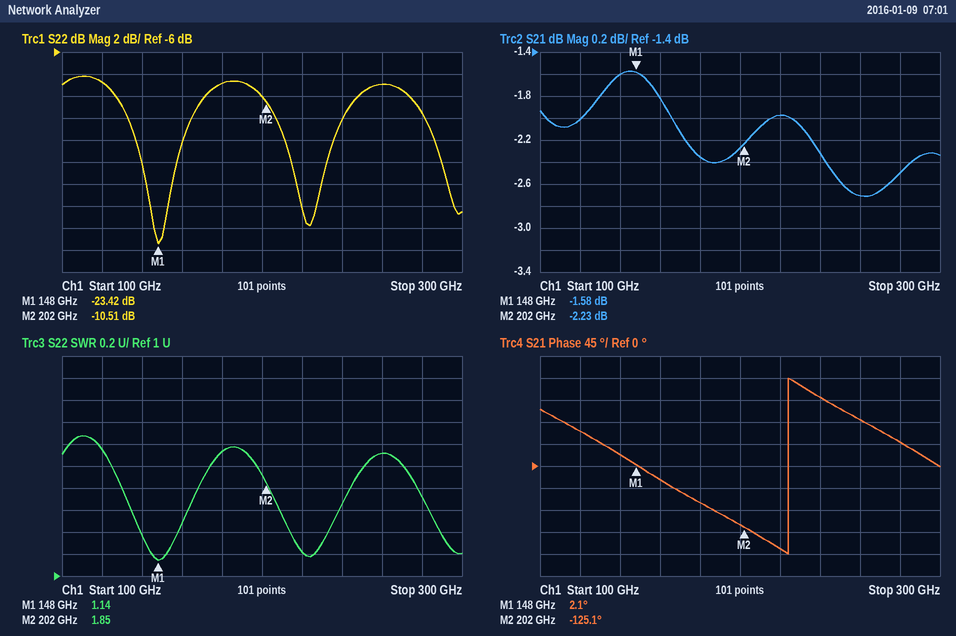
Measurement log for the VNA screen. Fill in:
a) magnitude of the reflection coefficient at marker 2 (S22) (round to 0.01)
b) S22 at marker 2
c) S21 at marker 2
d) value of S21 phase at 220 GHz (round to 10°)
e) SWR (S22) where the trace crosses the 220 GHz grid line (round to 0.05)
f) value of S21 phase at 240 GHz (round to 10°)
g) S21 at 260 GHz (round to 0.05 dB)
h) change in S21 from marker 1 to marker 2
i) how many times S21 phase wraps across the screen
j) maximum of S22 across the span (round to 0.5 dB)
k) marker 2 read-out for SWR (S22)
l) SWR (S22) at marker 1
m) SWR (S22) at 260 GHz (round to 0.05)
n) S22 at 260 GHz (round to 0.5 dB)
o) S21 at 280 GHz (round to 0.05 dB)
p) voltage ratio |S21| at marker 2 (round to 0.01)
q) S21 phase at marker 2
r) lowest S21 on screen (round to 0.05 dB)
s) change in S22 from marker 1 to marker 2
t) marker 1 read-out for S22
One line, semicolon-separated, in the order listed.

0.30; -10.51 dB; -2.23 dB; -170°; 1.20; 140°; -2.70 dB; -0.65 dB; 1; -8.0 dB; 1.85; 1.14; 2.10; -9.0 dB; -2.50 dB; 0.77; -125.1°; -2.70 dB; 12.91 dB; -23.42 dB
